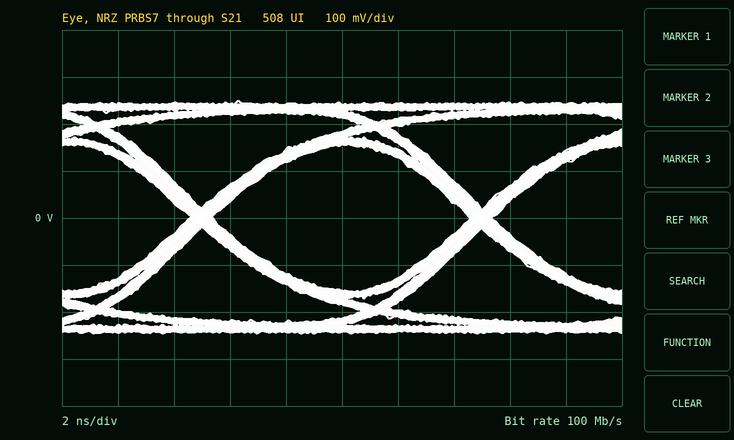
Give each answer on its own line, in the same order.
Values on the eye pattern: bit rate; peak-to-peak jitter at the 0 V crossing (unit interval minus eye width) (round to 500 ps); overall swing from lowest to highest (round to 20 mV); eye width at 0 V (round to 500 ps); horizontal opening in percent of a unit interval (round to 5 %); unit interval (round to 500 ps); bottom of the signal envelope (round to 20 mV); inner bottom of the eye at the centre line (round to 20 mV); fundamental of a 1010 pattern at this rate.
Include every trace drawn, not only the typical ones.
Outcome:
100 Mb/s
1.0 ns
500 mV
9.0 ns
90 %
10.0 ns
-240 mV
-160 mV
50 MHz
